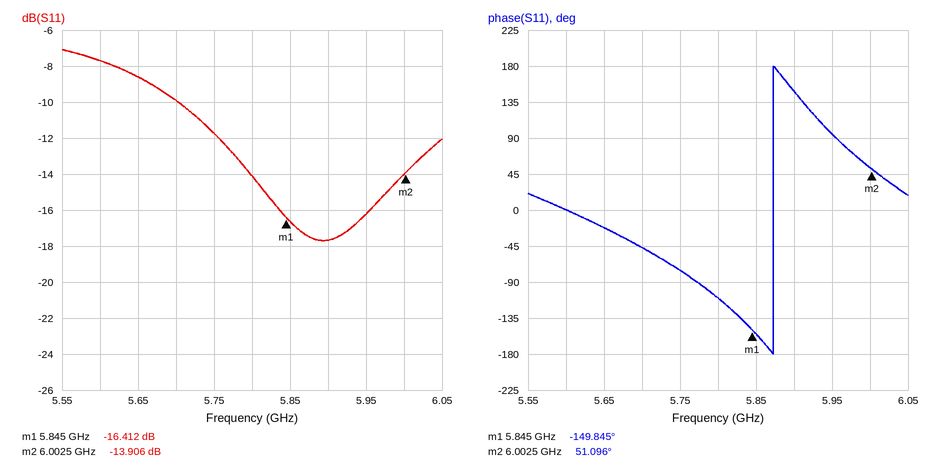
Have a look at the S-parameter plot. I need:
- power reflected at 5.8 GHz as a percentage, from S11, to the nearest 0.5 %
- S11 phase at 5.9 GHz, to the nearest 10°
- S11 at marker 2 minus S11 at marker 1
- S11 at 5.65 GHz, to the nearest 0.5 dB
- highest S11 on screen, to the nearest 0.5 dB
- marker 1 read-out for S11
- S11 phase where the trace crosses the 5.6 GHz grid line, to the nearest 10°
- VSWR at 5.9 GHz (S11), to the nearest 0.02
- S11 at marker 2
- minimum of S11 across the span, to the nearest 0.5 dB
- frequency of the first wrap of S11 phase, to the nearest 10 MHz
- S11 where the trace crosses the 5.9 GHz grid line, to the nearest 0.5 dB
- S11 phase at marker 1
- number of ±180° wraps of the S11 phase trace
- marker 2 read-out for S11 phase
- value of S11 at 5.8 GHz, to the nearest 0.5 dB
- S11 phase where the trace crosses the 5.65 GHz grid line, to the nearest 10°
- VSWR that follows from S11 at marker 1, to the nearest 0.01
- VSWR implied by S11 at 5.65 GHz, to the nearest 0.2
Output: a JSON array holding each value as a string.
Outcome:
["4.0 %", "150°", "2.506 dB", "-8.5 dB", "-7.0 dB", "-16.412 dB", "0°", "1.30", "-13.906 dB", "-17.5 dB", "5.87 GHz", "-17.5 dB", "-149.845°", "1", "51.096°", "-14.0 dB", "-20°", "1.36", "2.2"]
